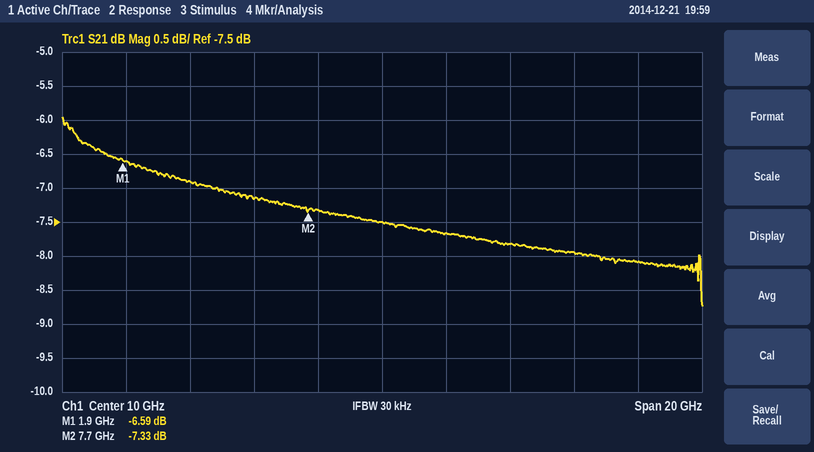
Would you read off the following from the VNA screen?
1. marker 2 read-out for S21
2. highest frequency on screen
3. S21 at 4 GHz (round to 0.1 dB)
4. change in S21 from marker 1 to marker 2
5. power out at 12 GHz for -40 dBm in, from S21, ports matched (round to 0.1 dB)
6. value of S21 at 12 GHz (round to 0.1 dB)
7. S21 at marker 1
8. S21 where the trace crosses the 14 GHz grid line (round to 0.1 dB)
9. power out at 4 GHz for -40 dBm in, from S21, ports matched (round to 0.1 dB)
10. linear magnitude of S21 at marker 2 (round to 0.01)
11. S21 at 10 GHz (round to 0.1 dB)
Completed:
-7.33 dB
20 GHz
-6.9 dB
-0.74 dB
-47.7 dBm
-7.7 dB
-6.59 dB
-7.8 dB
-46.9 dBm
0.43
-7.5 dB
